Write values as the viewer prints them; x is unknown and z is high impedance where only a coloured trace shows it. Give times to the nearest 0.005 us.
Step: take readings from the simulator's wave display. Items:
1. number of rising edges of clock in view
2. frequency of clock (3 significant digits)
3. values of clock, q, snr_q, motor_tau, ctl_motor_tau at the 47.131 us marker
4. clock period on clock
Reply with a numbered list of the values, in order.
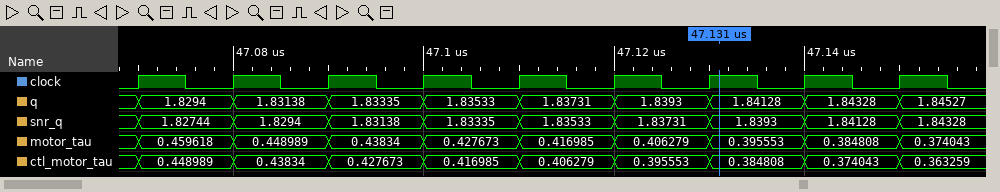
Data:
1. 9
2. 100 MHz
3. clock=1, q=1.84128, snr_q=1.8393, motor_tau=0.395553, ctl_motor_tau=0.384808
4. 0.01 us
